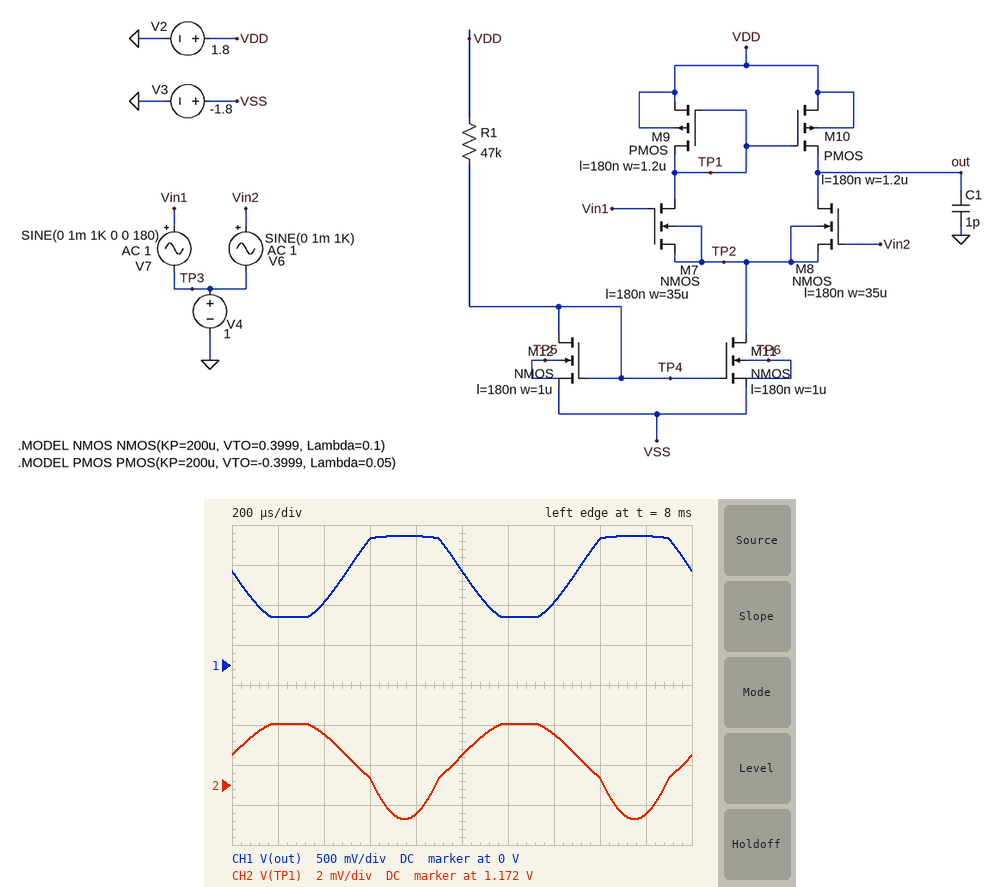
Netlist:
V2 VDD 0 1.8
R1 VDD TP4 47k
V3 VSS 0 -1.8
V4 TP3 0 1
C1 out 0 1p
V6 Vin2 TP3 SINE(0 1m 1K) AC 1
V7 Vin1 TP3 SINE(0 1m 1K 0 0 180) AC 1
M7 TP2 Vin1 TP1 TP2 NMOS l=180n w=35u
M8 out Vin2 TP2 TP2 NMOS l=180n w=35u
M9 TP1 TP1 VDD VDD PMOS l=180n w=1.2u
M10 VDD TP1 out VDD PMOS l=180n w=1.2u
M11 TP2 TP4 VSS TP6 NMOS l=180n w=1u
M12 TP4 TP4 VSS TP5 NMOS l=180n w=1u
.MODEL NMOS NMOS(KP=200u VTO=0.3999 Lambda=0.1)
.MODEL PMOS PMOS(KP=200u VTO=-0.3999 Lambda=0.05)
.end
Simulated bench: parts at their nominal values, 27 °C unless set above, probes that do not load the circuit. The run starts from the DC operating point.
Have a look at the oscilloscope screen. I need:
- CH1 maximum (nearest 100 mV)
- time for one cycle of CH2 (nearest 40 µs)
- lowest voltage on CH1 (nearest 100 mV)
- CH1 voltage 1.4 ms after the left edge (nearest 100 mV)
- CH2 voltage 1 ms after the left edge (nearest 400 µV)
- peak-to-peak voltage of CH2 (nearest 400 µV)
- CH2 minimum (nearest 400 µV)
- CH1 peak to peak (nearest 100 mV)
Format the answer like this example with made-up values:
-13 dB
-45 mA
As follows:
1.6 V
1.00 ms
600 mV
800 mV
1.1736 V
4.8 mV
1.1704 V
1.0 V
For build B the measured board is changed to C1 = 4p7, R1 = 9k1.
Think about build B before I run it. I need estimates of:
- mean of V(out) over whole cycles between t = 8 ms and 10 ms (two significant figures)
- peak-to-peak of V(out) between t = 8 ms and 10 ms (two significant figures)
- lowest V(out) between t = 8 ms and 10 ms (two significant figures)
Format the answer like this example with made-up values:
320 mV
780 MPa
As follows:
930 mV
630 mV
620 mV
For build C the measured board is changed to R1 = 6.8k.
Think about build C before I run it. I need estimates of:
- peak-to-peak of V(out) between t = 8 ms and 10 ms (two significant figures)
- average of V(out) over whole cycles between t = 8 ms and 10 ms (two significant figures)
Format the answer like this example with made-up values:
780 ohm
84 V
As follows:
550 mV
870 mV
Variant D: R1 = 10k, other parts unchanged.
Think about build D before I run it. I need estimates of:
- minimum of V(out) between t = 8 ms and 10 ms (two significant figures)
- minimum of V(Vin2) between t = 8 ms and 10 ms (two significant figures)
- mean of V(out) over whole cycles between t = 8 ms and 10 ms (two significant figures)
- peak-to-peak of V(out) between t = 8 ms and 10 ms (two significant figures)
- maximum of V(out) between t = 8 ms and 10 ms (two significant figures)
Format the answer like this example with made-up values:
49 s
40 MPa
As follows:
620 mV
1.0 V
950 mV
660 mV
1.3 V
